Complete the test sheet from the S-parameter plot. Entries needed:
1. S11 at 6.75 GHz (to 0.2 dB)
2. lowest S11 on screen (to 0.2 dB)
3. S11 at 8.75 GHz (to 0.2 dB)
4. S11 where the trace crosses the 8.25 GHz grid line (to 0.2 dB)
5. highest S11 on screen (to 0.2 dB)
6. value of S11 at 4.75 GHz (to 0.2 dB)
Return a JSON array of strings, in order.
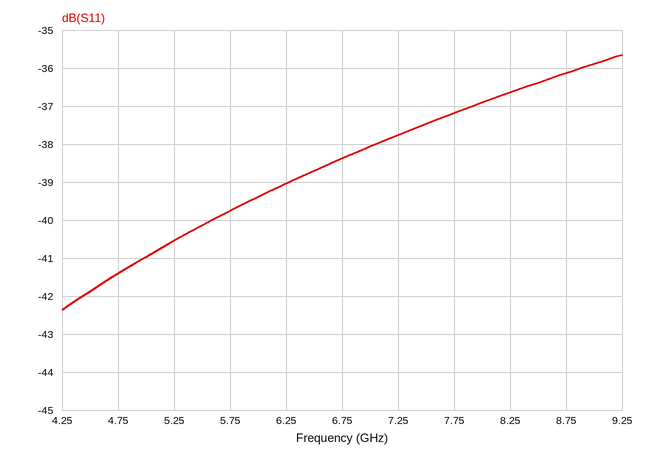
["-38.4 dB", "-42.4 dB", "-36.2 dB", "-36.6 dB", "-35.6 dB", "-41.4 dB"]
